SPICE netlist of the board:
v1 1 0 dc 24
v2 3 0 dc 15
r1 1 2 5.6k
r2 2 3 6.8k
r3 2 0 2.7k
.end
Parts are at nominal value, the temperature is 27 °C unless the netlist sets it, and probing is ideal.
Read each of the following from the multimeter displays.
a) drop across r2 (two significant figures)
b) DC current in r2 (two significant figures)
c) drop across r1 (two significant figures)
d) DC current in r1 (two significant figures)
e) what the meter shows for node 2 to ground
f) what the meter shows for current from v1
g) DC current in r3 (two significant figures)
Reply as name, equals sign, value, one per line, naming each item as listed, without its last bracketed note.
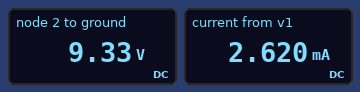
drop across r2 = 5.7 V
DC current in r2 = 830 µA
drop across r1 = 15 V
DC current in r1 = 2.6 mA
what the meter shows for node 2 to ground = 9.33 V
what the meter shows for current from v1 = 2.620 mA
DC current in r3 = 3.5 mA
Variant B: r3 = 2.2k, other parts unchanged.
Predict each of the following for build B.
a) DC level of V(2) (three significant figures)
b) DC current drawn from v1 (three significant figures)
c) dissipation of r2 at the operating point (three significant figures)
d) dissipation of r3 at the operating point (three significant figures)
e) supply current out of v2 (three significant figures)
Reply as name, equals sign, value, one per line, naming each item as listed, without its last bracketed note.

DC level of V(2) = 8.32 V
DC current drawn from v1 = 2.80 mA
dissipation of r2 at the operating point = 6.56 mW
dissipation of r3 at the operating point = 31.5 mW
supply current out of v2 = 982 µA
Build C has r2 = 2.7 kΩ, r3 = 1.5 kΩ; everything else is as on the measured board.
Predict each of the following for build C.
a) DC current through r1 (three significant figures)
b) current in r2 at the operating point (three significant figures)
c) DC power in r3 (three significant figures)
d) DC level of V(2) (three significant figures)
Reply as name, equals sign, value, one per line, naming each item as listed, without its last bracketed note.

DC current through r1 = 2.84 mA
current in r2 at the operating point = 2.56 mA
DC power in r3 = 43.7 mW
DC level of V(2) = 8.10 V
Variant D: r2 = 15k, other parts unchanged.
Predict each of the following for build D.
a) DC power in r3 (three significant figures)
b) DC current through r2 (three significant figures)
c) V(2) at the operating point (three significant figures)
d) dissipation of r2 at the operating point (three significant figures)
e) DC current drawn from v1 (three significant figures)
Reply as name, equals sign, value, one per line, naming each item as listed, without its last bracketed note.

DC power in r3 = 27.3 mW
DC current through r2 = 428 µA
V(2) at the operating point = 8.59 V
dissipation of r2 at the operating point = 2.74 mW
DC current drawn from v1 = 2.75 mA
